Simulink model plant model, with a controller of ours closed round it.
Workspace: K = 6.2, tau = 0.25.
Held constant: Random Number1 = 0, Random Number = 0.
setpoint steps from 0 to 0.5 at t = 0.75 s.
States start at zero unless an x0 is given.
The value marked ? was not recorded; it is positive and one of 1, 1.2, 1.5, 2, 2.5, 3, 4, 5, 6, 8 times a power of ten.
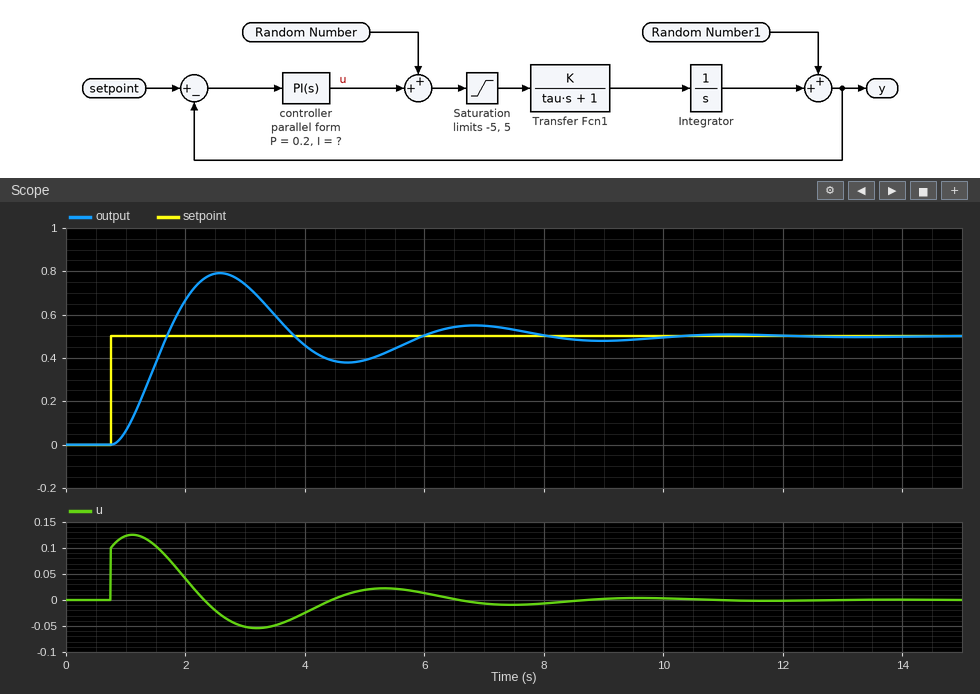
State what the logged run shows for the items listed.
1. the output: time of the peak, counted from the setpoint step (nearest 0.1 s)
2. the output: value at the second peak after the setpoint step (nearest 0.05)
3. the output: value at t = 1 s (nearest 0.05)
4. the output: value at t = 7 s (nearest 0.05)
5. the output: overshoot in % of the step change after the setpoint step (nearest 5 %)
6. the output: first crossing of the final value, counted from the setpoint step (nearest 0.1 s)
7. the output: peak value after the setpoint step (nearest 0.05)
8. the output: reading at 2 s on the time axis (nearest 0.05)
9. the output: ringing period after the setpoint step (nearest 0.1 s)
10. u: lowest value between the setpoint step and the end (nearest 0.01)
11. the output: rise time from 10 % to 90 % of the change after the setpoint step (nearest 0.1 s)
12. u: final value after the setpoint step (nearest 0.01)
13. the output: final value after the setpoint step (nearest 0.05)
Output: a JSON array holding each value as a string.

["1.8 s", "0.55", "0.05", "0.55", "60 %", "0.9 s", "0.80", "0.65", "4.3 s", "-0.05", "0.6 s", "0.00", "0.50"]
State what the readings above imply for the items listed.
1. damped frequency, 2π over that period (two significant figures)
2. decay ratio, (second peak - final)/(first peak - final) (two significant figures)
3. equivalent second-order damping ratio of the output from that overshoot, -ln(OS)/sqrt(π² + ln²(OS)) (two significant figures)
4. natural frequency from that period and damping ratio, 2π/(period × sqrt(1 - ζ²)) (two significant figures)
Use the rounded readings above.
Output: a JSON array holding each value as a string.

["1.5 rad/s", "0.17", "0.16", "1.5 rad/s"]
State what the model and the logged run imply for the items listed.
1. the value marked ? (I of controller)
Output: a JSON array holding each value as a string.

["0.3"]
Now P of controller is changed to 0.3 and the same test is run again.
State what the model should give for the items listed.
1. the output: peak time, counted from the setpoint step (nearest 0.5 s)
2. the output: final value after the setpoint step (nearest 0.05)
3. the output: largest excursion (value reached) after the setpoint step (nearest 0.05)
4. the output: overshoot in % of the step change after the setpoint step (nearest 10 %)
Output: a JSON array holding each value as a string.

["1.5 s", "0.50", "0.70", "40 %"]
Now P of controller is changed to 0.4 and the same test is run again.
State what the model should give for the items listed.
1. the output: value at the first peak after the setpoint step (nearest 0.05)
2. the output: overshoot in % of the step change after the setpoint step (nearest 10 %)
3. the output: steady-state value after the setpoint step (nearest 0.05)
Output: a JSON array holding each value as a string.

["0.70", "40 %", "0.50"]
